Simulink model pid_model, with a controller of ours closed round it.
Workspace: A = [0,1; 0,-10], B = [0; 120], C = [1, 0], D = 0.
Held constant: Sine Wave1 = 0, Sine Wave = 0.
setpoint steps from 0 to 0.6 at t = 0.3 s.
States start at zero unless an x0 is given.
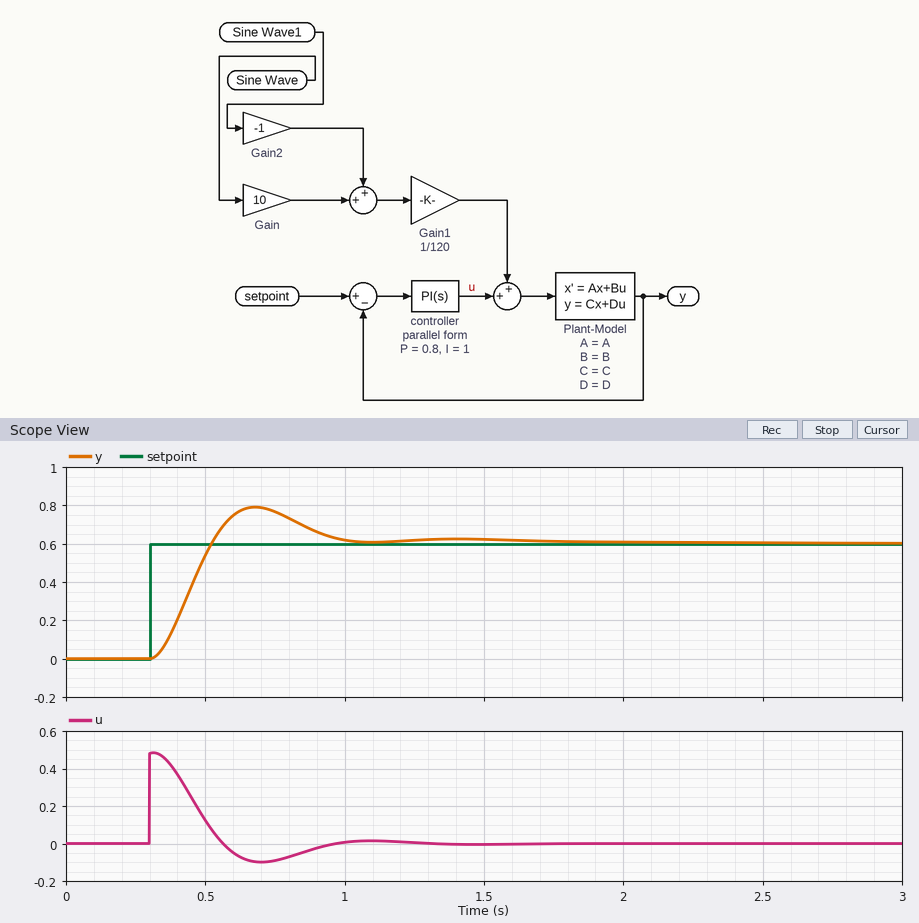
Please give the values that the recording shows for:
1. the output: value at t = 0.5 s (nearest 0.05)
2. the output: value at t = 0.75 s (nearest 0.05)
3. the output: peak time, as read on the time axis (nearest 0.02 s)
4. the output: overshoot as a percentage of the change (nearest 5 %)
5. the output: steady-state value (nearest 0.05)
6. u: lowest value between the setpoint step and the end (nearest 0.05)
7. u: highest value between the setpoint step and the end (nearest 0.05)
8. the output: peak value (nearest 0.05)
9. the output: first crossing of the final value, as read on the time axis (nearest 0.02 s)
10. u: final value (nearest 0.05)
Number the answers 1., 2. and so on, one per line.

1. 0.55
2. 0.75
3. 0.68 s
4. 30 %
5. 0.60
6. -0.10
7. 0.50
8. 0.80
9. 0.52 s
10. 0.00
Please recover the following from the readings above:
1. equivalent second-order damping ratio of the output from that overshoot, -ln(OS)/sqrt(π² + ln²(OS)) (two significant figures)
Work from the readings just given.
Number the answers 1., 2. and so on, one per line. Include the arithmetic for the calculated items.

1. ln(0.3) = -1.204; 1.204 / sqrt(9.870 + 1.450) = 0.36
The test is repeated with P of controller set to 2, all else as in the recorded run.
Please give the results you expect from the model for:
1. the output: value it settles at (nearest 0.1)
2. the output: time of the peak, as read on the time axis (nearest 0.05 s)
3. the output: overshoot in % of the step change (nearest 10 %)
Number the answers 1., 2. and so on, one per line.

1. 0.6
2. 0.50 s
3. 40 %
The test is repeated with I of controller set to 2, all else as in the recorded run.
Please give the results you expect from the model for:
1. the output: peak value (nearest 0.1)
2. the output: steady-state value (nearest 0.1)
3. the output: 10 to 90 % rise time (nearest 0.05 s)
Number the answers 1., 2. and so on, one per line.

1. 0.9
2. 0.6
3. 0.15 s
